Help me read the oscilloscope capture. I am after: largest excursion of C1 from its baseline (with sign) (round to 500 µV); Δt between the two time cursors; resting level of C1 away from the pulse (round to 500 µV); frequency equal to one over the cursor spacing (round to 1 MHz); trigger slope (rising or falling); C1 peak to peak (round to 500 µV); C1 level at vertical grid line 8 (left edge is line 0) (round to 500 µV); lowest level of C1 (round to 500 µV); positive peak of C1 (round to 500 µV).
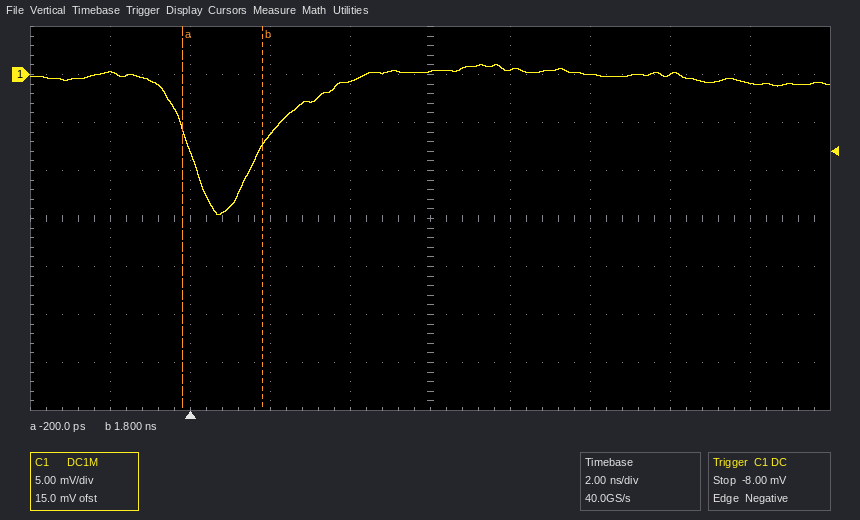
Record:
-14.5 mV
2.0 ns
0.0 mV
500 MHz
falling
15.5 mV
0.0 mV
-14.5 mV
1.0 mV
